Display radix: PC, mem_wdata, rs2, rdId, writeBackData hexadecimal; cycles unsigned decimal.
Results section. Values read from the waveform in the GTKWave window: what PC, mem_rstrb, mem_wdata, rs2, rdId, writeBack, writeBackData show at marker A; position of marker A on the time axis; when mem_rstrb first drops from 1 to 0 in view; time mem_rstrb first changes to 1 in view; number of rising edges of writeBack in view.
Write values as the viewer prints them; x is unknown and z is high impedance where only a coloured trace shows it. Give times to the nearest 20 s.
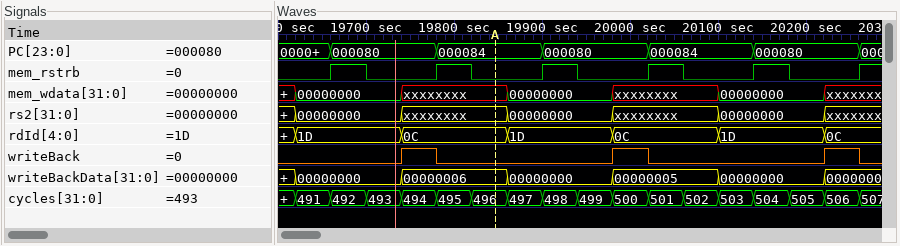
PC=000084, mem_rstrb=0, mem_wdata=xxxxxxxx, rs2=xxxxxxxx, rdId=0C, writeBack=0, writeBackData=00000006
19840 s
19700 s
19660 s
3
